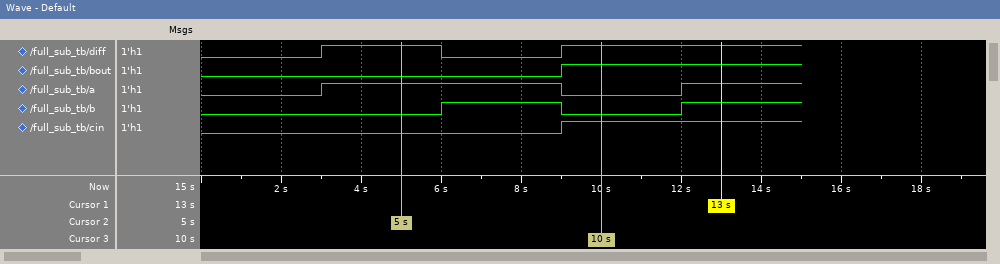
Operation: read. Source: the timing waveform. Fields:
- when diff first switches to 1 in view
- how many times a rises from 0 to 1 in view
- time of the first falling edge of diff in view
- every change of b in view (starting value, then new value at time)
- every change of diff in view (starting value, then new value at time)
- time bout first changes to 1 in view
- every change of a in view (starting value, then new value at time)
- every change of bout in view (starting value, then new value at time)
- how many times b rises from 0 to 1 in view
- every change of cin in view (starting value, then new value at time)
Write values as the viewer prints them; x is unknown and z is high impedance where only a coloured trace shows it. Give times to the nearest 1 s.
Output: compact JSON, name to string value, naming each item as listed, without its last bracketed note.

{"when diff first switches to 1 in view": "3 s", "how many times a rises from 0 to 1 in view": "2", "time of the first falling edge of diff in view": "6 s", "every change of b in view": "0, 1 at 6 s, 0 at 9 s, 1 at 12 s", "every change of diff in view": "0, 1 at 3 s, 0 at 6 s, 1 at 9 s", "time bout first changes to 1 in view": "9 s", "every change of a in view": "0, 1 at 3 s, 0 at 9 s, 1 at 12 s", "every change of bout in view": "0, 1 at 9 s", "how many times b rises from 0 to 1 in view": "2", "every change of cin in view": "0, 1 at 9 s"}
